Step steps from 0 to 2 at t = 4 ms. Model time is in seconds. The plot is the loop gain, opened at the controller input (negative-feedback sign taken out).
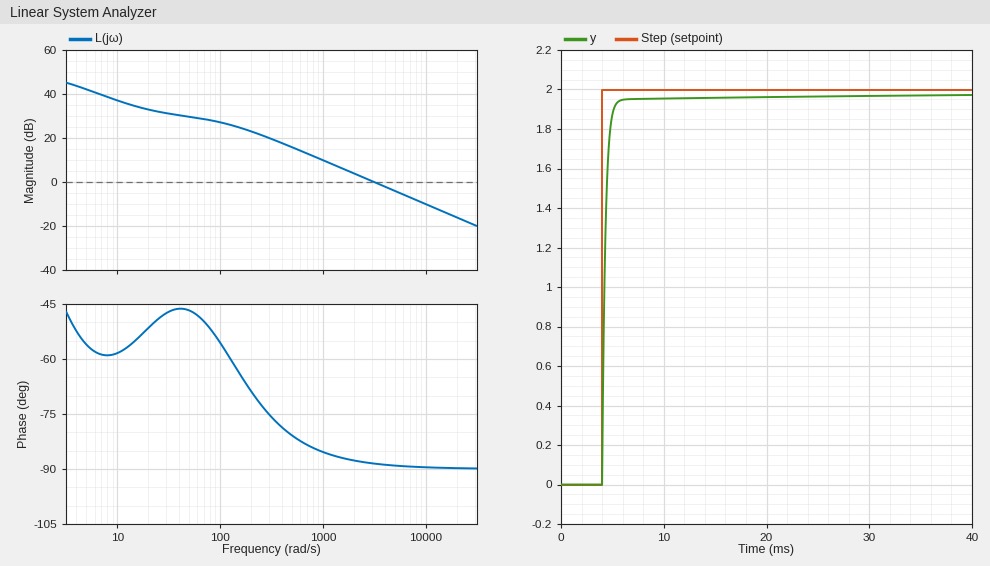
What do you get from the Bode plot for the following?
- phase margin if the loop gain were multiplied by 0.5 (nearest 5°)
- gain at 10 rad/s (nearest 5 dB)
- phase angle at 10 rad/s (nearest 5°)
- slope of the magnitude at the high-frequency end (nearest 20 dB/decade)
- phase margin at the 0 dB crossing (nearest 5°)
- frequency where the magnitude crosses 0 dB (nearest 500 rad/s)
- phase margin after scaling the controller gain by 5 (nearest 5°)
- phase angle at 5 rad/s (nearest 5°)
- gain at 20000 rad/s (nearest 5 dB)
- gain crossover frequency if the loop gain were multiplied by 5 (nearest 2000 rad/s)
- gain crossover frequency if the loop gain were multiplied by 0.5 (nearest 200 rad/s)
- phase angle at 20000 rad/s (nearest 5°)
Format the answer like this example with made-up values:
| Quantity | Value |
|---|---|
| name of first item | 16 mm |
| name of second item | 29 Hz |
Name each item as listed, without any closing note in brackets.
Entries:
| Quantity | Value |
|---|---|
| phase margin if the loop gain were multiplied by 0.5 | 95° |
| gain at 10 rad/s | 35 dB |
| phase angle at 10 rad/s | -60° |
| slope of the magnitude at the high-frequency end | -20 dB/decade |
| phase margin at the 0 dB crossing | 90° |
| frequency where the magnitude crosses 0 dB | 3000 rad/s |
| phase margin after scaling the controller gain by 5 | 90° |
| phase angle at 5 rad/s | -55° |
| gain at 20000 rad/s | -15 dB |
| gain crossover frequency if the loop gain were multiplied by 5 | 16000 rad/s |
| gain crossover frequency if the loop gain were multiplied by 0.5 | 1600 rad/s |
| phase angle at 20000 rad/s | -90° |
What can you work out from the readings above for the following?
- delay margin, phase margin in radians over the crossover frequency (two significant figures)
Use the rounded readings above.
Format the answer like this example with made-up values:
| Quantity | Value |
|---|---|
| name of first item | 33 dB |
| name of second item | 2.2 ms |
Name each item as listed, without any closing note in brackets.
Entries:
| Quantity | Value |
|---|---|
| delay margin, phase margin in radians over the crossover frequency | 0.00052 s |
